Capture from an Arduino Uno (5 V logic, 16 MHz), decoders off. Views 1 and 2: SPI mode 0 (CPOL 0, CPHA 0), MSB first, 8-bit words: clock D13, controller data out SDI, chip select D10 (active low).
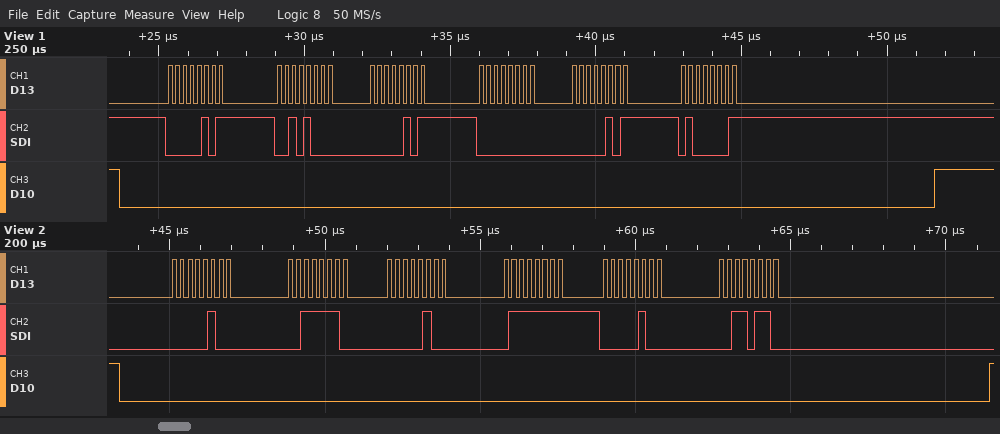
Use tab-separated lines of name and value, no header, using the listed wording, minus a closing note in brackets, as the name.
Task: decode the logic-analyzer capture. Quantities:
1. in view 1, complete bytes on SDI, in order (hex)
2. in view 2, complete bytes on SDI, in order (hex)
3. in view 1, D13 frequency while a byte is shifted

in view 1, complete bytes on SDI, in order	05 28 05 00 05 41
in view 2, complete bytes on SDI, in order	04 3E 04 7F 04 36
in view 1, D13 frequency while a byte is shifted	4 MHz
